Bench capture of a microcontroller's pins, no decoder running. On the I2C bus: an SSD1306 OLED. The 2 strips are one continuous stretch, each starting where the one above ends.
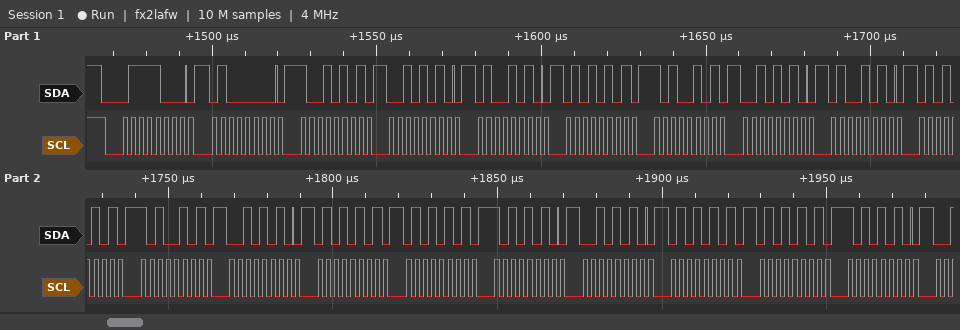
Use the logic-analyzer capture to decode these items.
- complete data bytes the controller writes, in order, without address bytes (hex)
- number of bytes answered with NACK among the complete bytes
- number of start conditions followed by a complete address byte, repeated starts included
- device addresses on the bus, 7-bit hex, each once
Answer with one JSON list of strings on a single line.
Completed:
["40 95 2A 4A 55 A5 2A 4A 55 A5 2A 55 55 AA 2A 55 55 AA", "0", "1", "0x3C"]
